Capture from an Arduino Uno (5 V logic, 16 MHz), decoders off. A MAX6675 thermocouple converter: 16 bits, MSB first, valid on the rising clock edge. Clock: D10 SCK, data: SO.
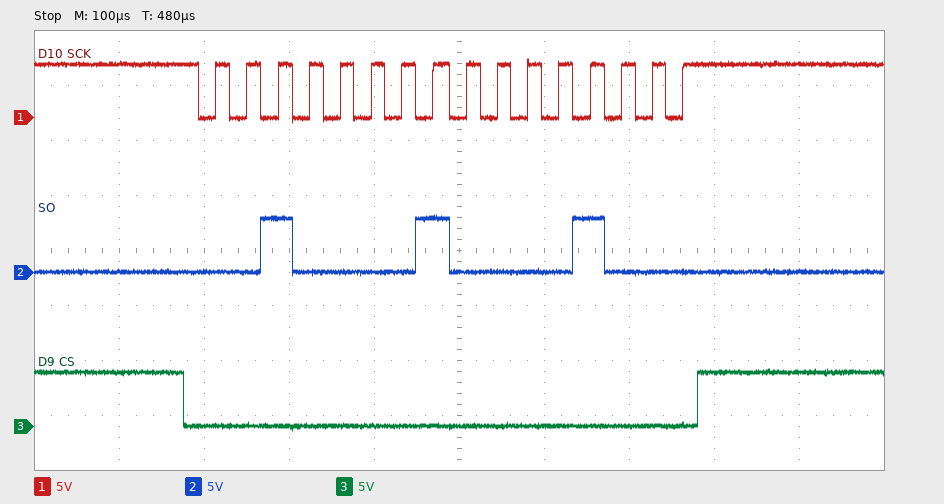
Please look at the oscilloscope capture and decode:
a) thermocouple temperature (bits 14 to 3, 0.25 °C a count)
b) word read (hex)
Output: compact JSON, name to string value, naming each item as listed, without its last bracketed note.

{"thermocouple temperature": "264.25 °C", "word read": "0x2108"}
